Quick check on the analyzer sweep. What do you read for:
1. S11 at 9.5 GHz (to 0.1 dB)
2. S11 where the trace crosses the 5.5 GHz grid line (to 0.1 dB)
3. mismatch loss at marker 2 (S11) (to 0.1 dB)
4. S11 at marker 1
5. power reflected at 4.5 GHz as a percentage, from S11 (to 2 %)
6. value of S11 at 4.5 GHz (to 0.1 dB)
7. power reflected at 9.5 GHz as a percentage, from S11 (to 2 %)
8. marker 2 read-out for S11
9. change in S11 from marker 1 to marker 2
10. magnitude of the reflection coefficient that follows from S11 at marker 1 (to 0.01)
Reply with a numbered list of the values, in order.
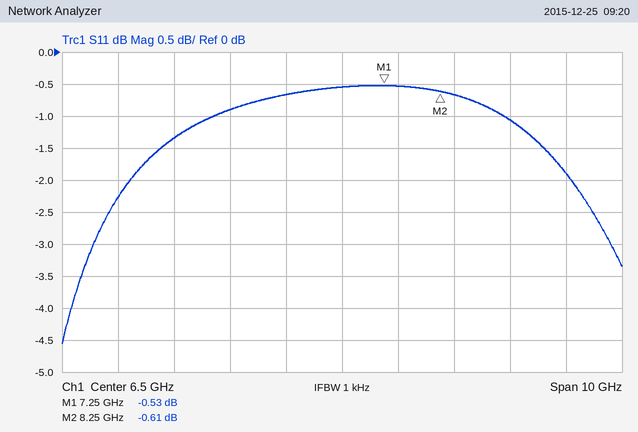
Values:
1. -1.1 dB
2. -0.7 dB
3. 8.8 dB
4. -0.53 dB
5. 82 %
6. -0.9 dB
7. 78 %
8. -0.61 dB
9. -0.08 dB
10. 0.94
